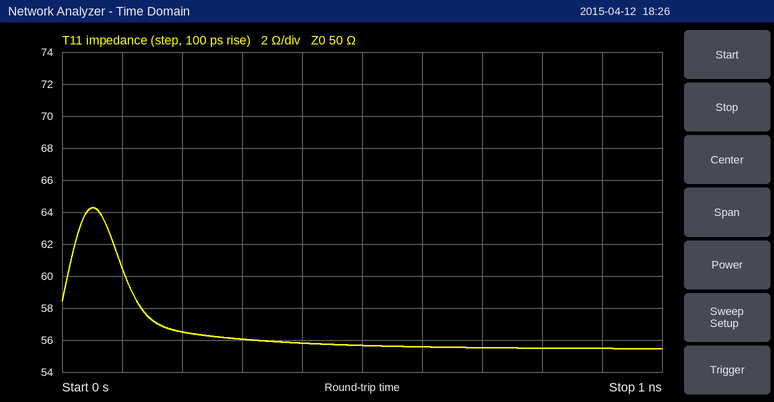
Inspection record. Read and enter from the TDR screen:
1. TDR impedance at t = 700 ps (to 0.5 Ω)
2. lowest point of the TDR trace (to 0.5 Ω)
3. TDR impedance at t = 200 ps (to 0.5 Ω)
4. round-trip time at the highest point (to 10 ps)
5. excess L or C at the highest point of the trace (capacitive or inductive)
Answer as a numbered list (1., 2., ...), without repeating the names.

1. 55.5 Ω
2. 55.5 Ω
3. 56.5 Ω
4. 50 ps
5. inductive
